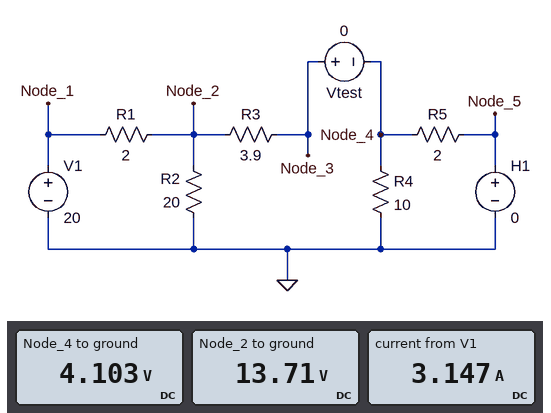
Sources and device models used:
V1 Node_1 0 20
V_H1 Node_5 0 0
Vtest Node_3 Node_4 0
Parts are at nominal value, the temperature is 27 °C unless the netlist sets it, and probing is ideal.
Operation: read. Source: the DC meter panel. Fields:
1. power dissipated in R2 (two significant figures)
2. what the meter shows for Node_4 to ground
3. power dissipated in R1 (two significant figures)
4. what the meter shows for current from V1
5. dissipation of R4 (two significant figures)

9.4 W
4.103 V
20 W
3.147 A
1.7 W
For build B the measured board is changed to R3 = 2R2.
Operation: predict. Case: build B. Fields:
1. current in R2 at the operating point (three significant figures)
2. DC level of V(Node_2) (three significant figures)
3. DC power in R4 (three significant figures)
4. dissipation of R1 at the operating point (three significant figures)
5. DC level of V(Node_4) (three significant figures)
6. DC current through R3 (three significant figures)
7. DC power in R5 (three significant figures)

618 mA
12.4 V
2.84 W
29.1 W
5.33 V
3.20 A
14.2 W
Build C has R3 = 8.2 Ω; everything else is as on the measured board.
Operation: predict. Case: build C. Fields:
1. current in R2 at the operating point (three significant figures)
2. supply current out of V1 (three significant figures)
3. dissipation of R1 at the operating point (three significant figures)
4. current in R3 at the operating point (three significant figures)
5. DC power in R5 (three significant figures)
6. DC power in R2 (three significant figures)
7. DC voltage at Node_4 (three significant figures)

768 mA
2.32 A
10.8 W
1.56 A
3.36 W
11.8 W
2.59 V
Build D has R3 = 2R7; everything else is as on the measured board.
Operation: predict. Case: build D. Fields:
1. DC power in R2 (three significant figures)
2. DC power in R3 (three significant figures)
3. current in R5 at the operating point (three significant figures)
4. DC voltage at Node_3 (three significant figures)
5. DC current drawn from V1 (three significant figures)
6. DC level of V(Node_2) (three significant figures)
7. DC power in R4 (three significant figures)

8.24 W
23.3 W
2.45 A
4.90 V
3.58 A
12.8 V
2.40 W
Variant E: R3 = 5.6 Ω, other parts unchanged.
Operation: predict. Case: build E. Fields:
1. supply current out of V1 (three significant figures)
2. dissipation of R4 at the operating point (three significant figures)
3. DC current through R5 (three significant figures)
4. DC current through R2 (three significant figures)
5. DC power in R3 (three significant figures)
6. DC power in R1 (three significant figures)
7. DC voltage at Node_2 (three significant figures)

2.73 A
1.11 W
1.67 A
727 mA
22.4 W
14.9 W
14.5 V
